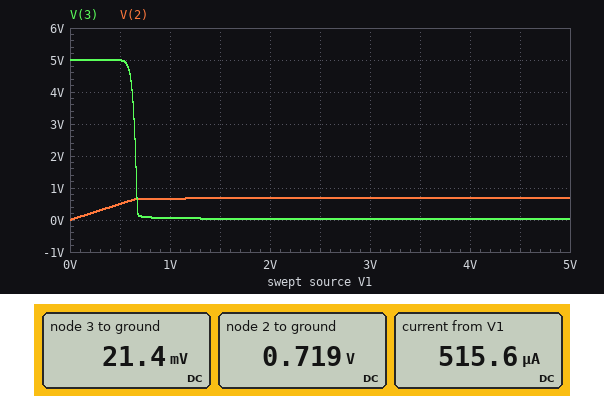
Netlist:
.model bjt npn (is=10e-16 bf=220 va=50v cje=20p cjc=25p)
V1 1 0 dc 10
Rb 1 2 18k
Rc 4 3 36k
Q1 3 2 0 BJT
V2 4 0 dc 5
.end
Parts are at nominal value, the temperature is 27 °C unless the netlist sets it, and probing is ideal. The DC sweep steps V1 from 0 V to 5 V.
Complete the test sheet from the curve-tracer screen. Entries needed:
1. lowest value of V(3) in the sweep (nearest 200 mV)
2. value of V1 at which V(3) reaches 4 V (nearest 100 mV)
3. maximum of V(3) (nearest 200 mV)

0 V
600 mV
5.0 V
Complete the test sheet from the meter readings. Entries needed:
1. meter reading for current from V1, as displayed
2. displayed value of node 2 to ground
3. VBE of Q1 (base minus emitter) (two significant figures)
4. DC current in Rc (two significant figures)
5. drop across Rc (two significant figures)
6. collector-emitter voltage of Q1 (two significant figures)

515.6 µA
0.719 V
720 mV
140 µA
5.0 V
21 mV
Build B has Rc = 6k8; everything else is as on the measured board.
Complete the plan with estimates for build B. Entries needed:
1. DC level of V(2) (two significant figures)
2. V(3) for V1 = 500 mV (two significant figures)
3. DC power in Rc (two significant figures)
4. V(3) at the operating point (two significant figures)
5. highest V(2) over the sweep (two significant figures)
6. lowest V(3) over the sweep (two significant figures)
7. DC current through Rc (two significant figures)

730 mV
5.0 V
3.6 mW
32 mV
720 mV
43 mV
730 µA
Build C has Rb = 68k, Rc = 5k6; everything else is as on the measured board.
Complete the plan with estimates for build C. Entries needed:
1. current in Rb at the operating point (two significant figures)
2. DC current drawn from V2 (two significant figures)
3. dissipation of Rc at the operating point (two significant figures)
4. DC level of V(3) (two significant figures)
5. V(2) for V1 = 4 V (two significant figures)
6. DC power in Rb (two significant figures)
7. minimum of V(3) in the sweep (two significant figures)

140 µA
880 µA
4.4 mW
56 mV
710 mV
1.3 mW
74 mV
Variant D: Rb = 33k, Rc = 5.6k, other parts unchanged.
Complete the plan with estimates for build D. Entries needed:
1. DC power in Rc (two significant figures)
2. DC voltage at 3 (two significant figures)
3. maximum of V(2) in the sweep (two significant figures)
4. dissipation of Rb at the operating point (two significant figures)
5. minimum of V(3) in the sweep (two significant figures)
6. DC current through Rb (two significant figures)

4.4 mW
43 mV
720 mV
2.6 mW
57 mV
280 µA
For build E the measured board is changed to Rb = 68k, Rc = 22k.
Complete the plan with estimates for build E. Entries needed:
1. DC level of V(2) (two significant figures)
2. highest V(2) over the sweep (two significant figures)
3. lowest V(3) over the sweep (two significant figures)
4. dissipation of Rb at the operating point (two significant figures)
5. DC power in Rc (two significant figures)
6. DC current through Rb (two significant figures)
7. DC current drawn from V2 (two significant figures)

700 mV
690 mV
45 mV
1.3 mW
1.1 mW
140 µA
230 µA
